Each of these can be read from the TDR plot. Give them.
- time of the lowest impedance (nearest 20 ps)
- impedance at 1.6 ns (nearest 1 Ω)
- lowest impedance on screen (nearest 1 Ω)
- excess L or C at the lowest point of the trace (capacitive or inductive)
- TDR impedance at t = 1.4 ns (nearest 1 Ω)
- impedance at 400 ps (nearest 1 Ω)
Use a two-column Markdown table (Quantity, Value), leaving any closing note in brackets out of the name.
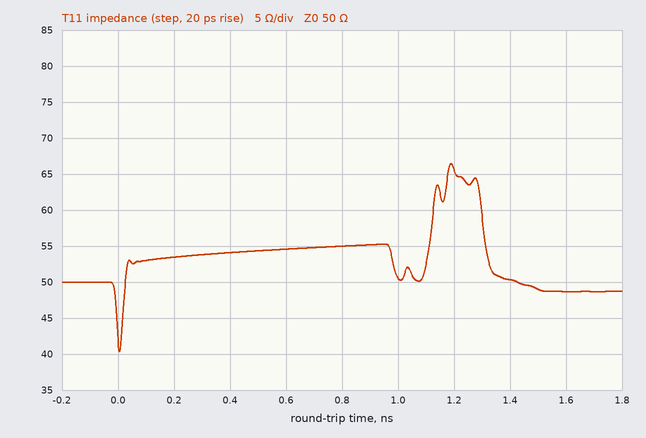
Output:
| Quantity | Value |
|---|---|
| time of the lowest impedance | 0 ps |
| impedance at 1.6 ns | 49 Ω |
| lowest impedance on screen | 40 Ω |
| excess L or C at the lowest point of the trace | capacitive |
| TDR impedance at t = 1.4 ns | 50 Ω |
| impedance at 400 ps | 54 Ω |
